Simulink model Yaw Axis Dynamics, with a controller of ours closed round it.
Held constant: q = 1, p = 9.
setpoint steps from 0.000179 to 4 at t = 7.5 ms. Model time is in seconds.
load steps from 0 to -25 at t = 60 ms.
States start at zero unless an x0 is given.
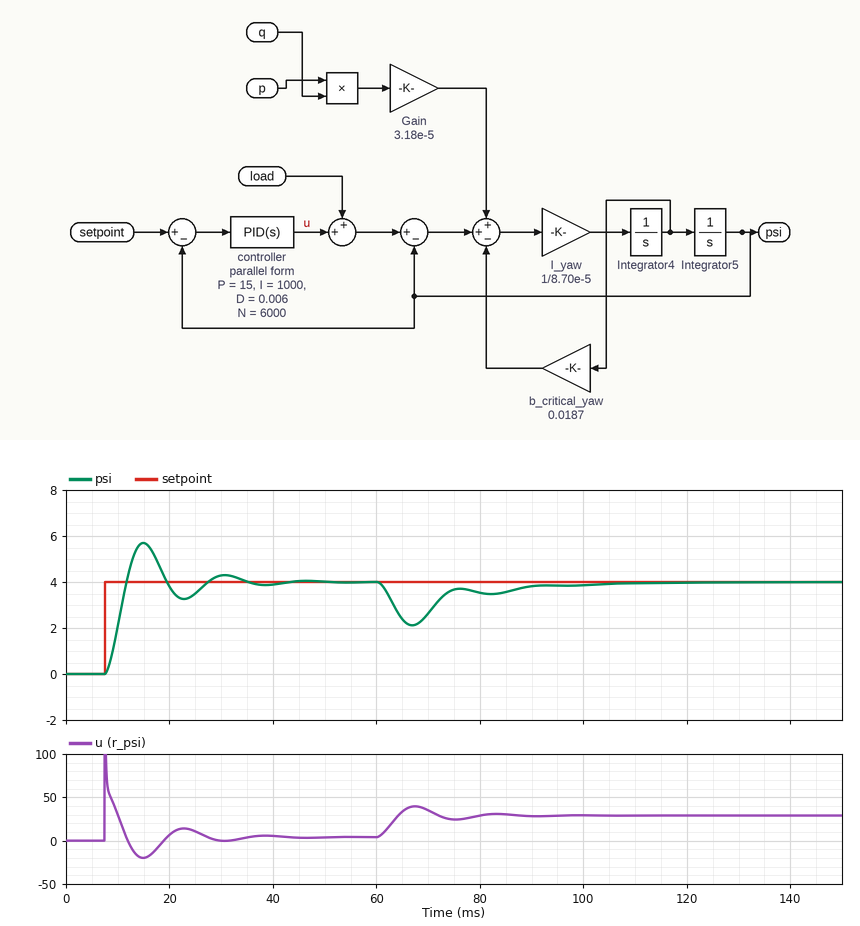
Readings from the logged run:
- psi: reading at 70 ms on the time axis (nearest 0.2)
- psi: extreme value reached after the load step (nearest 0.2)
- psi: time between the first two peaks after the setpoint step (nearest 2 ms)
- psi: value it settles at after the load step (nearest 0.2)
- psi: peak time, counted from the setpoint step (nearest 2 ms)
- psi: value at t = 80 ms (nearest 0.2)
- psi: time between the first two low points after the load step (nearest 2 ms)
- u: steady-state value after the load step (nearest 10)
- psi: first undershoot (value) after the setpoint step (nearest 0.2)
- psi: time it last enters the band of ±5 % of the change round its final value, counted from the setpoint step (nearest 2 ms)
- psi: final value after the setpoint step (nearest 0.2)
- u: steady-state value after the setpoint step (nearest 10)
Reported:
2.6
2.2
16 ms
4.0
8 ms
3.6
16 ms
30
3.2
26 ms
4.0
0
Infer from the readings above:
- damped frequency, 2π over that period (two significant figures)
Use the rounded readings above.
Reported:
0.39 rad/ms
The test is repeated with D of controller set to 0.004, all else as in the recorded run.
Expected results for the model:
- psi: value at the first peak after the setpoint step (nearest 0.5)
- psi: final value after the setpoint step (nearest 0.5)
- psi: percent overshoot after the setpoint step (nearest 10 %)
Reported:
6.0
4.0
50 %
